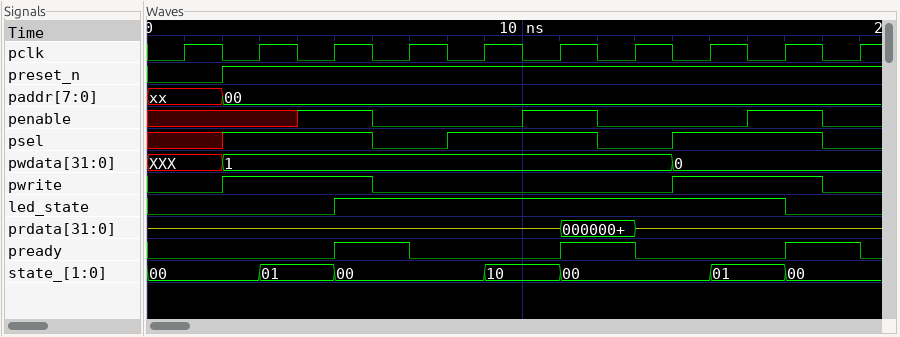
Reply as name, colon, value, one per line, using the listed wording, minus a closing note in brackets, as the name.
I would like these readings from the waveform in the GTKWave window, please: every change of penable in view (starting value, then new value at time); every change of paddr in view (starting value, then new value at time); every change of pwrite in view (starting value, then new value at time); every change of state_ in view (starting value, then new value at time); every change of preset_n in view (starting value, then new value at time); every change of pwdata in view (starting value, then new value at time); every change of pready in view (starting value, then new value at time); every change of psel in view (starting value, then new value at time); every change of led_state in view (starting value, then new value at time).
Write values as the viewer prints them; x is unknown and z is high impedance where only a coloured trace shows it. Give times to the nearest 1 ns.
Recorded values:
every change of penable in view: x, 1 at 4 ns, 0 at 6 ns, 1 at 10 ns, 0 at 12 ns, 1 at 16 ns, 0 at 18 ns
every change of paddr in view: xx, 00 at 2 ns
every change of pwrite in view: 0, 1 at 2 ns, 0 at 6 ns, 1 at 14 ns, 0 at 18 ns
every change of state_ in view: 00, 01 at 3 ns, 00 at 5 ns, 10 at 9 ns, 00 at 11 ns, 01 at 15 ns, 00 at 17 ns
every change of preset_n in view: 0, 1 at 2 ns
every change of pwdata in view: XXX, 1 at 2 ns, 0 at 14 ns
every change of pready in view: 0, 1 at 5 ns, 0 at 7 ns, 1 at 11 ns, 0 at 13 ns, 1 at 17 ns, 0 at 19 ns
every change of psel in view: x, 1 at 2 ns, 0 at 6 ns, 1 at 8 ns, 0 at 12 ns, 1 at 14 ns, 0 at 18 ns
every change of led_state in view: 0, 1 at 5 ns, 0 at 17 ns
